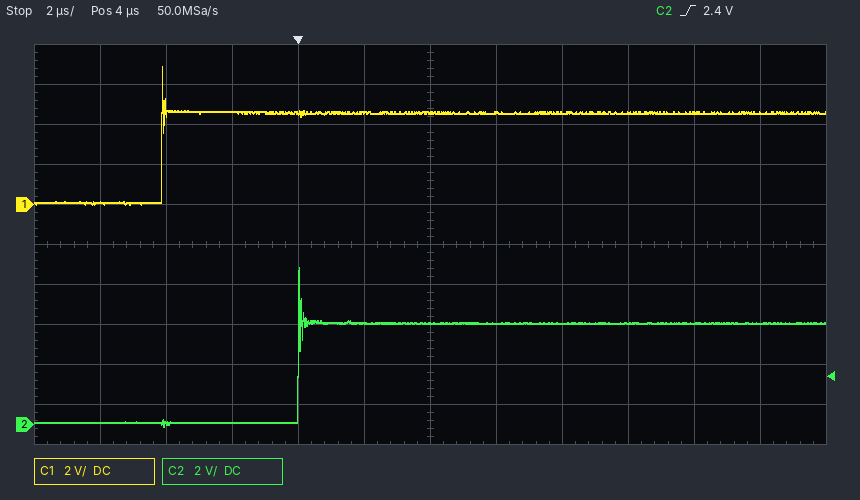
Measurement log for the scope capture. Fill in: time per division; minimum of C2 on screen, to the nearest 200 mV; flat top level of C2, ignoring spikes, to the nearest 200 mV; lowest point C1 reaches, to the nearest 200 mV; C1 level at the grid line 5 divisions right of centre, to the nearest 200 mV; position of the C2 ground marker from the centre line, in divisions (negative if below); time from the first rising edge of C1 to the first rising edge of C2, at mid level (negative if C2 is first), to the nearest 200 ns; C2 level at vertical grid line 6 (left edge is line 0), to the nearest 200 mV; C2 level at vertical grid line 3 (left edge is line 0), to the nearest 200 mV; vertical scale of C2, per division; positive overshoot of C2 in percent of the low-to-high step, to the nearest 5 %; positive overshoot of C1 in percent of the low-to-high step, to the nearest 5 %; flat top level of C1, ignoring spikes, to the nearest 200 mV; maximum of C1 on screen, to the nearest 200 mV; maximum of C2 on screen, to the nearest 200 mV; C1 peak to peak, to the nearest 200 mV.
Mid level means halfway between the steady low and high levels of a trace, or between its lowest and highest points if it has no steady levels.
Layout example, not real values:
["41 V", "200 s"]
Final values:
["2 µs", "0.0 V", "5.0 V", "0.0 V", "4.6 V", "-4.5 div", "+4.2 µs", "5.0 V", "0.0 V", "2 V", "55 %", "50 %", "4.6 V", "6.8 V", "7.8 V", "6.8 V"]
